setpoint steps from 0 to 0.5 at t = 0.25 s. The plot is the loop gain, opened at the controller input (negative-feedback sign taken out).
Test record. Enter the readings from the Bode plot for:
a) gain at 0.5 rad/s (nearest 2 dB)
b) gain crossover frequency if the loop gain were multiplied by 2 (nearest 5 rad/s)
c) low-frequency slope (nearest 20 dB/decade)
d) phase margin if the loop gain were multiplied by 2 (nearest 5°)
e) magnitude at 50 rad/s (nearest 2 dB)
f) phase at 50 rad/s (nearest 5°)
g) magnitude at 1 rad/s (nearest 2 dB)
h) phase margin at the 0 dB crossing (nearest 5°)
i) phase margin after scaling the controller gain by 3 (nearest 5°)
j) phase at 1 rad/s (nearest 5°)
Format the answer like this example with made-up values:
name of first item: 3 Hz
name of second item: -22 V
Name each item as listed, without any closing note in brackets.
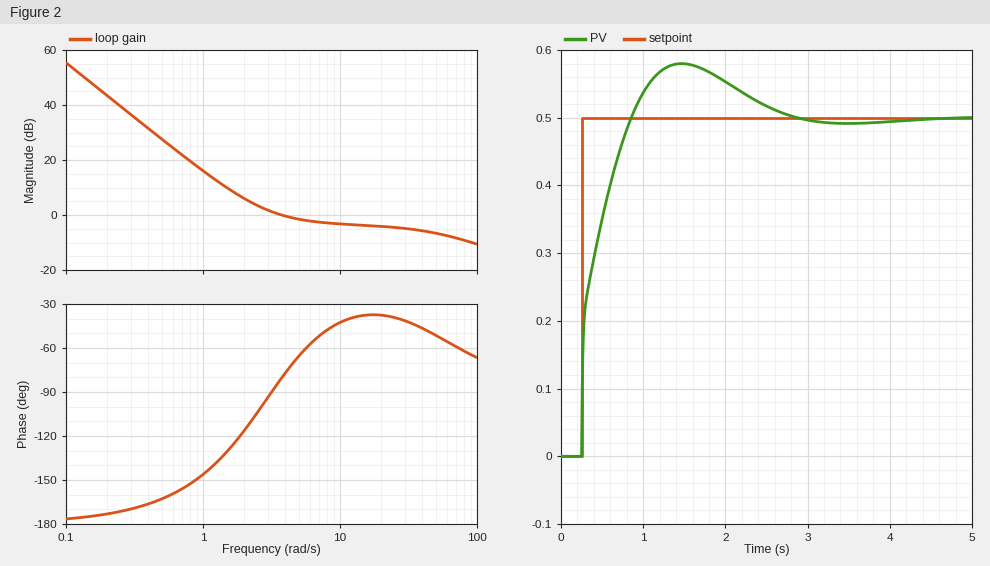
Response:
gain at 0.5 rad/s: 28 dB
gain crossover frequency if the loop gain were multiplied by 2: 45 rad/s
low-frequency slope: -40 dB/decade
phase margin if the loop gain were multiplied by 2: 130°
magnitude at 50 rad/s: -6 dB
phase at 50 rad/s: -50°
magnitude at 1 rad/s: 16 dB
phase margin at the 0 dB crossing: 100°
phase margin after scaling the controller gain by 3: 115°
phase at 1 rad/s: -145°
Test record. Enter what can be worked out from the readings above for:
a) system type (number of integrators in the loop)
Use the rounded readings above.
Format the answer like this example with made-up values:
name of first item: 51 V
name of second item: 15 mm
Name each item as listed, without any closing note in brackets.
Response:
system type: 2
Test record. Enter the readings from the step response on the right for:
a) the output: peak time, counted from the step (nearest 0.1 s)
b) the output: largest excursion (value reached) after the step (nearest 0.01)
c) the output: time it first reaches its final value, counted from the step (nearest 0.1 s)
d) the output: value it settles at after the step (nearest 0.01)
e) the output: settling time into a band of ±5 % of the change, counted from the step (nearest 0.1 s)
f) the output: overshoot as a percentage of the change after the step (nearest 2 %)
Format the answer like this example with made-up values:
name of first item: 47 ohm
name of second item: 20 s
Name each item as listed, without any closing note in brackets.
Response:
the output: peak time, counted from the step: 1.2 s
the output: largest excursion (value reached) after the step: 0.58
the output: time it first reaches its final value, counted from the step: 0.6 s
the output: value it settles at after the step: 0.50
the output: settling time into a band of ±5 % of the change, counted from the step: 2.1 s
the output: overshoot as a percentage of the change after the step: 16 %
